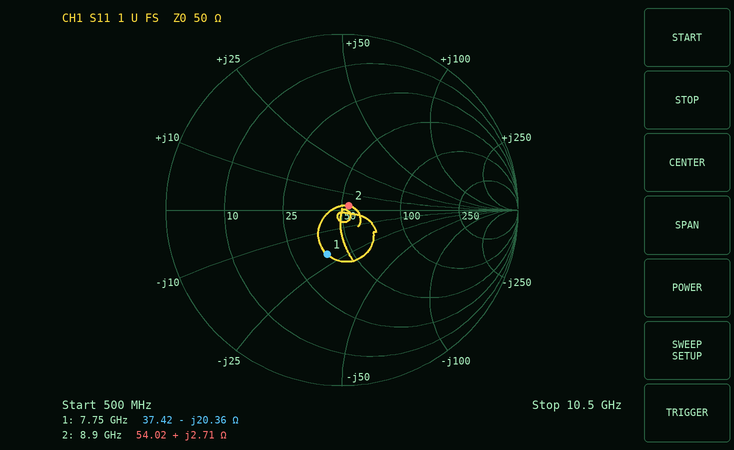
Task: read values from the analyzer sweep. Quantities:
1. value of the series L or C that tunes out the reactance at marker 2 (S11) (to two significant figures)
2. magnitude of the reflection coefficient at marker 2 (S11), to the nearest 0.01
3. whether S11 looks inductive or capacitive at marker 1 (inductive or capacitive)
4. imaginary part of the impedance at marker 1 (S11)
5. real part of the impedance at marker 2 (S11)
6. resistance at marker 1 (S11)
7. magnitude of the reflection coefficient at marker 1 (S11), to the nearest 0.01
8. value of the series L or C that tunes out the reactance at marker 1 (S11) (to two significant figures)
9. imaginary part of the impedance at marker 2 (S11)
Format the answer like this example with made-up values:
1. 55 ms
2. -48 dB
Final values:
1. 6.6 pF
2. 0.05
3. capacitive
4. -20.36 Ω
5. 54.02 Ω
6. 37.42 Ω
7. 0.27
8. 420 pH
9. +2.71 Ω
